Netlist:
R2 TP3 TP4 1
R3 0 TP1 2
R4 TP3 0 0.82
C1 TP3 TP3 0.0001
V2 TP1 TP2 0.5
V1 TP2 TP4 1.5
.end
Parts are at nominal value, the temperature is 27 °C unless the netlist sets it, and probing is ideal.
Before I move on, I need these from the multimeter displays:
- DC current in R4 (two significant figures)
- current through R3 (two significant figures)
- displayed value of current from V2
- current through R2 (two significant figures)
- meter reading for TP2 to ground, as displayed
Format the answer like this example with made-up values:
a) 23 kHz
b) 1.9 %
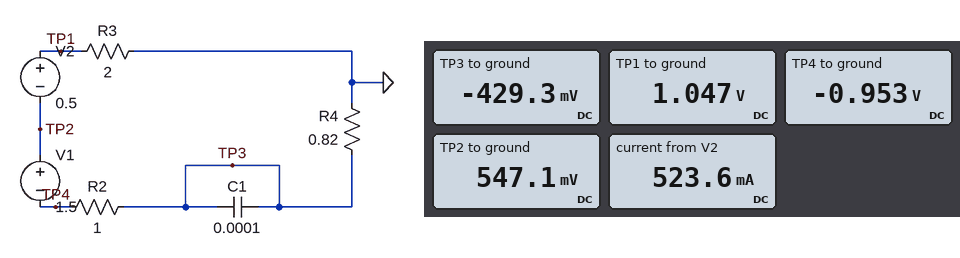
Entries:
a) 520 mA
b) 520 mA
c) 523.6 mA
d) 520 mA
e) 547.1 mV
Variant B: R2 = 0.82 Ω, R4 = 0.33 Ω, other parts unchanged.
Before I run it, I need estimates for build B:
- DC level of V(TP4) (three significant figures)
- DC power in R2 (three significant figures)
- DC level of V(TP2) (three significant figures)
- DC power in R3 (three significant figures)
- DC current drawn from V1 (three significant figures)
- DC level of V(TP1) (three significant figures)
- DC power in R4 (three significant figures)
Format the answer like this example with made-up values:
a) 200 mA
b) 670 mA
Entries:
a) -730 mV
b) 331 mW
c) 770 mV
d) 806 mW
e) 635 mA
f) 1.27 V
g) 133 mW
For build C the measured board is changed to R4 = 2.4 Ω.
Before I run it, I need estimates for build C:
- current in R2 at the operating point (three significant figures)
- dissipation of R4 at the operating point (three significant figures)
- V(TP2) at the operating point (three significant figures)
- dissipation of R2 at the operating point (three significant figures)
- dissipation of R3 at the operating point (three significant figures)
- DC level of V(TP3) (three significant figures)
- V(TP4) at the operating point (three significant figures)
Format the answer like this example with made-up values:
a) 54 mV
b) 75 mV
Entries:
a) 370 mA
b) 329 mW
c) 241 mV
d) 137 mW
e) 274 mW
f) -889 mV
g) -1.26 V
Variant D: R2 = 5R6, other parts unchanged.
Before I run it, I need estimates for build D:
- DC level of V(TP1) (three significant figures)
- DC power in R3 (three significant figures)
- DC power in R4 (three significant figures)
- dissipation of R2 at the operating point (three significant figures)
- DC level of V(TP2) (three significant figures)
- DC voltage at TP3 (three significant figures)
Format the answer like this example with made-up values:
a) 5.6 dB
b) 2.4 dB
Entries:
a) 475 mV
b) 113 mW
c) 46.3 mW
d) 316 mW
e) -24.9 mV
f) -195 mV
